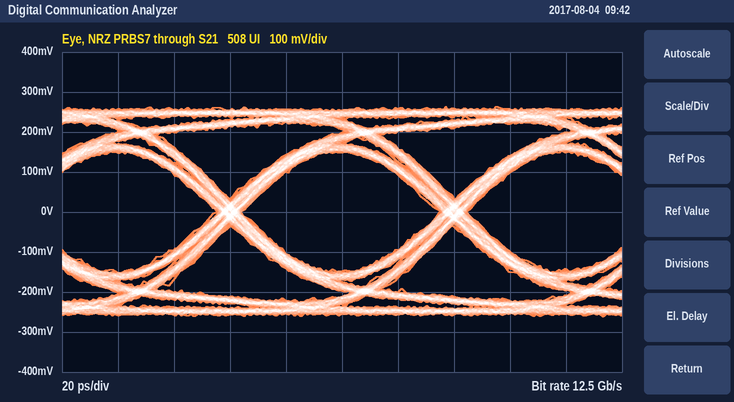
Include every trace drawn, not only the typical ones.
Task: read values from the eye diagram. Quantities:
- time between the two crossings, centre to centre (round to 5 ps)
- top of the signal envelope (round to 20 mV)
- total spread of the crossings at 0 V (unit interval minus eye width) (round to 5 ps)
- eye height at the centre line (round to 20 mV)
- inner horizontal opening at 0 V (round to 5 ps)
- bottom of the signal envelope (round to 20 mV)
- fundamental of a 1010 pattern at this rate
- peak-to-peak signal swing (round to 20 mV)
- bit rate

80 ps
260 mV
10 ps
300 mV
70 ps
-260 mV
6.25 GHz
520 mV
12.5 Gb/s
